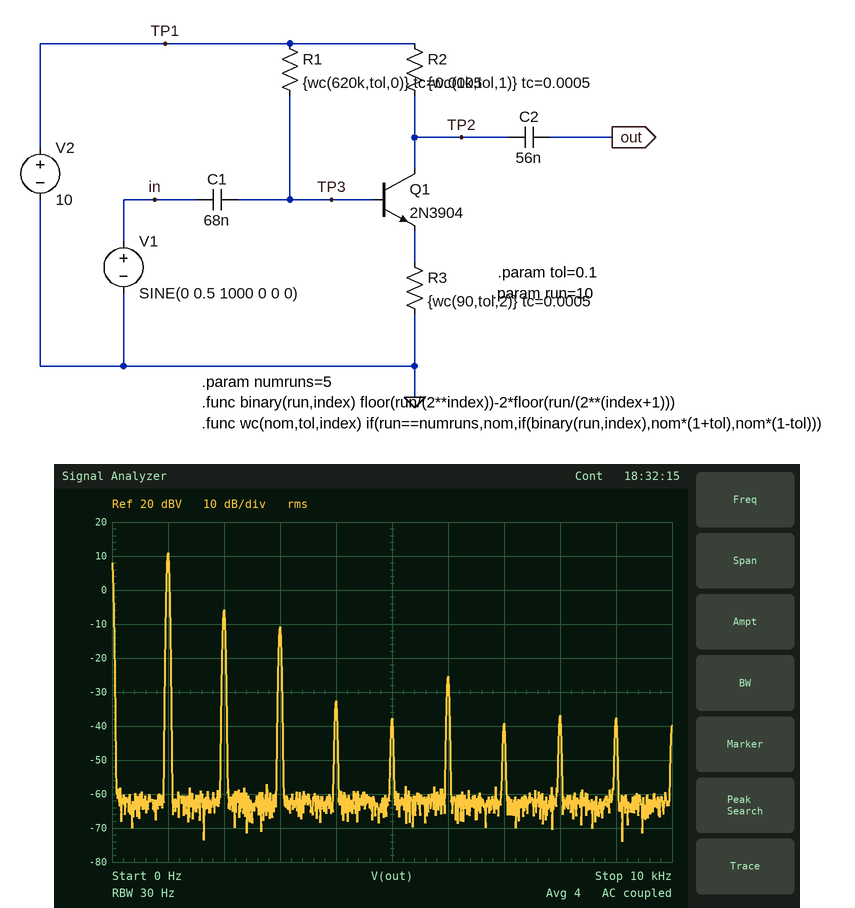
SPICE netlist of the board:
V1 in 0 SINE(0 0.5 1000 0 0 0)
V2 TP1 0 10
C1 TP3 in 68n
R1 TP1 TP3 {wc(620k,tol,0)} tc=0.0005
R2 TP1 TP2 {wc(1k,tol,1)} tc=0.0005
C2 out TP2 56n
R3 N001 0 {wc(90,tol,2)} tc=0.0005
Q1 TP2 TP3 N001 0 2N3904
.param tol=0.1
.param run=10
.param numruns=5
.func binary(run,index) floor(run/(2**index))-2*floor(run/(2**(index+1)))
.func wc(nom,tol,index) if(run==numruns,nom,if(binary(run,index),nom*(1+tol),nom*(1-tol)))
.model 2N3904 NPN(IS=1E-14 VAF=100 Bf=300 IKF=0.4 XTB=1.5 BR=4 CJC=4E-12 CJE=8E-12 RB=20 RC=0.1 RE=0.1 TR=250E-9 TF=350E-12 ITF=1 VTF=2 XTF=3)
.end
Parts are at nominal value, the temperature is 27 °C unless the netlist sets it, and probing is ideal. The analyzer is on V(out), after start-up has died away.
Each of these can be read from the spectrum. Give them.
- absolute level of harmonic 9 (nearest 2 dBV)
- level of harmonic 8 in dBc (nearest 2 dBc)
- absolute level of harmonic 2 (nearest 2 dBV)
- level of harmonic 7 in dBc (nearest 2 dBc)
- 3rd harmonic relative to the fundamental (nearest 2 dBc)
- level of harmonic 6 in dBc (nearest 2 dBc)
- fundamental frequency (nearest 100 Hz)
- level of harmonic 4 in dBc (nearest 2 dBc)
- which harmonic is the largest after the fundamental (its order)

-38 dBV
-48 dBc
-6 dBV
-50 dBc
-22 dBc
-36 dBc
1.0 kHz
-44 dBc
2
